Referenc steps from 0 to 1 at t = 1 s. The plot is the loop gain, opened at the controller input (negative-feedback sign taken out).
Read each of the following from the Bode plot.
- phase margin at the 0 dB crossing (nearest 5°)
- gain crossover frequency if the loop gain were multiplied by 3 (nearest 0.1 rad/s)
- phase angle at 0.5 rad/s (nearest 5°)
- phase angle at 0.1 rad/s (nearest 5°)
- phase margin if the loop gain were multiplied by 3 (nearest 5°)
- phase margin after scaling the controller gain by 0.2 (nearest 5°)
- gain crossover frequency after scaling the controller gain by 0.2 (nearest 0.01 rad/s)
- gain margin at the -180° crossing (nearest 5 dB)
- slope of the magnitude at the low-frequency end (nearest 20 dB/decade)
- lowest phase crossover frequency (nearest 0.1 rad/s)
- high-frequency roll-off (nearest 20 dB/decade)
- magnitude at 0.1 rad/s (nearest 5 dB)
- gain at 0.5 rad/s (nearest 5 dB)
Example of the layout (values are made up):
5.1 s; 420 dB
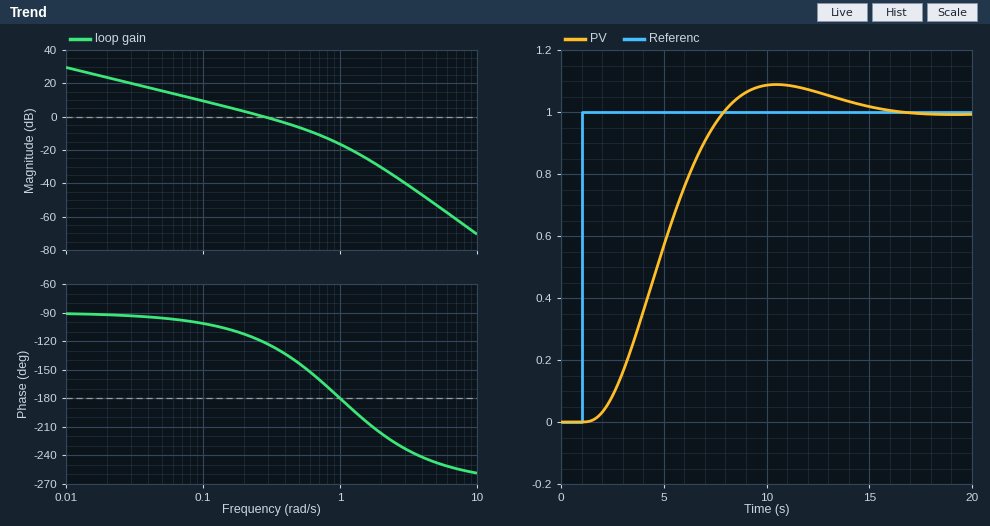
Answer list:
60°; 0.6 rad/s; -145°; -100°; 25°; 85°; 0.06 rad/s; 15 dB; -20 dB/decade; 1.0 rad/s; -60 dB/decade; 10 dB; -5 dB
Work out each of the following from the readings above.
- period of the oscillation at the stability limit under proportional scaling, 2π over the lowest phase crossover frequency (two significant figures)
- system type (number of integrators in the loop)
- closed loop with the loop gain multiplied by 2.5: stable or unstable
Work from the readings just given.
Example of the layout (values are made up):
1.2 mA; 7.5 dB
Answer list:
6.3 s; 1; stable
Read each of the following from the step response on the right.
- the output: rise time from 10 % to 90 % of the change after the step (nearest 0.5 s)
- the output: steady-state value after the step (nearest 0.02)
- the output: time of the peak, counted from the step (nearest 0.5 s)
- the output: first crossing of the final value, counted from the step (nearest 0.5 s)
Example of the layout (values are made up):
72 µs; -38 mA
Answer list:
4.5 s; 1.00; 9.5 s; 7.0 s
